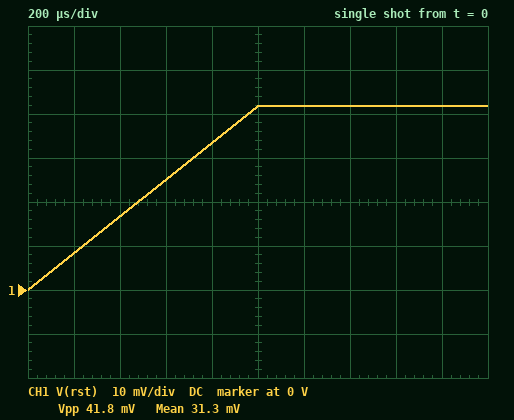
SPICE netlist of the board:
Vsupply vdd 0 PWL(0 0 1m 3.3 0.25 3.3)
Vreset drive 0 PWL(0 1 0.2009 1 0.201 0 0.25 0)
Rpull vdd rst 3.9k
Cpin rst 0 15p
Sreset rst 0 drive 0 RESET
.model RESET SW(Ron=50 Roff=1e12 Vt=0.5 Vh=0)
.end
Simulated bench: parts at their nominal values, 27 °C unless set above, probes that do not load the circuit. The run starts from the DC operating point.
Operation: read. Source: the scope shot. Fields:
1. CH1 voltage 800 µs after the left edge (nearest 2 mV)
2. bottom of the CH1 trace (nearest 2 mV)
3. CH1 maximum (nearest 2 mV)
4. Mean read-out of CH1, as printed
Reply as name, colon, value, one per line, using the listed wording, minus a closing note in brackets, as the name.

CH1 voltage 800 µs after the left edge: 34 mV
bottom of the CH1 trace: 0 V
CH1 maximum: 42 mV
Mean read-out of CH1, as printed: 31.3 mV
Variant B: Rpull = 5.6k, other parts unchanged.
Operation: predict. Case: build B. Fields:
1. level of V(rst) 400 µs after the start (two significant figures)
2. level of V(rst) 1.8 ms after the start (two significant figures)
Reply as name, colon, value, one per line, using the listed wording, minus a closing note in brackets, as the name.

level of V(rst) 400 µs after the start: 12 mV
level of V(rst) 1.8 ms after the start: 29 mV
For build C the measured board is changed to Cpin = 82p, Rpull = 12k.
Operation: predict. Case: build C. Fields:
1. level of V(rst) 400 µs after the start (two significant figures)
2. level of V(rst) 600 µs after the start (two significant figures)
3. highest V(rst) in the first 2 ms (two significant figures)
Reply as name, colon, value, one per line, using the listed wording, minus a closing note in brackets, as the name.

level of V(rst) 400 µs after the start: 5.5 mV
level of V(rst) 600 µs after the start: 8.2 mV
highest V(rst) in the first 2 ms: 14 mV
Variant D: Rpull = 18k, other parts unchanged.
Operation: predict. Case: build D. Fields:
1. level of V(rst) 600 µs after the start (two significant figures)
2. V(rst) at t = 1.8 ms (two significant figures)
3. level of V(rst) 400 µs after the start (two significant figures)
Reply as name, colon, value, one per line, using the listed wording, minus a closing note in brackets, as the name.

level of V(rst) 600 µs after the start: 5.5 mV
V(rst) at t = 1.8 ms: 9.1 mV
level of V(rst) 400 µs after the start: 3.7 mV
